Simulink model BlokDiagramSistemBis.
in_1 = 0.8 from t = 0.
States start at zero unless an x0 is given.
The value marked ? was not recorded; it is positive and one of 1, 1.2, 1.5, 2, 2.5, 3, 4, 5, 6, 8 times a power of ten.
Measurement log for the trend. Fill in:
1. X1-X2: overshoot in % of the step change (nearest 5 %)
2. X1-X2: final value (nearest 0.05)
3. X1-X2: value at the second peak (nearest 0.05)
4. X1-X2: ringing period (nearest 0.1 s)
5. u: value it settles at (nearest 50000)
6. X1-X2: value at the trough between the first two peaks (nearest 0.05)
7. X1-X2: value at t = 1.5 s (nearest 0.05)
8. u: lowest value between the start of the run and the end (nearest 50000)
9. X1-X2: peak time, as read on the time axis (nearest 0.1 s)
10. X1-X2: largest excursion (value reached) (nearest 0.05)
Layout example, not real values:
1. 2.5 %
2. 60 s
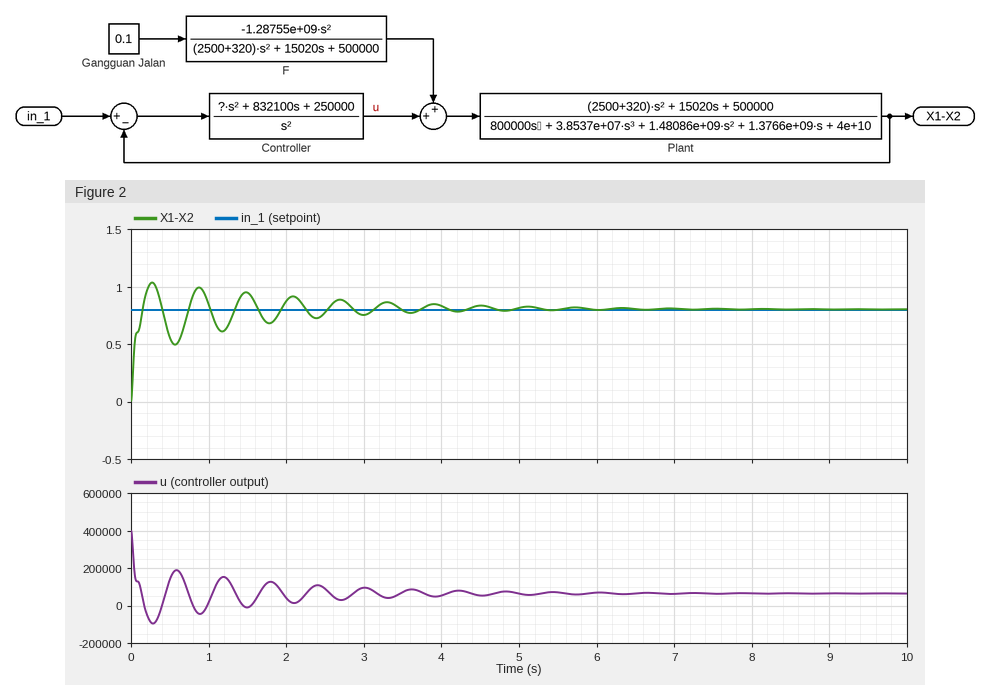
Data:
1. 30 %
2. 0.80
3. 1.00
4. 0.6 s
5. 50000
6. 0.50
7. 0.95
8. -100000
9. 0.3 s
10. 1.05
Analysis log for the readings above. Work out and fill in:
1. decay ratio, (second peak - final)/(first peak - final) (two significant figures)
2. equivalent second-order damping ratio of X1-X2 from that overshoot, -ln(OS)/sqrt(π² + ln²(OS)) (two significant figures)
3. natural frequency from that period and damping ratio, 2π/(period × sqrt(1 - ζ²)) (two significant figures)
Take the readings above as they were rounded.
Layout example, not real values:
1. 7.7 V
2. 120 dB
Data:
1. 0.80
2. 0.36
3. 11 rad/s
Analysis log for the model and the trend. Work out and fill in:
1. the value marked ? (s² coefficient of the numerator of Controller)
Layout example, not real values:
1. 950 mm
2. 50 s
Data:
1. 500000
